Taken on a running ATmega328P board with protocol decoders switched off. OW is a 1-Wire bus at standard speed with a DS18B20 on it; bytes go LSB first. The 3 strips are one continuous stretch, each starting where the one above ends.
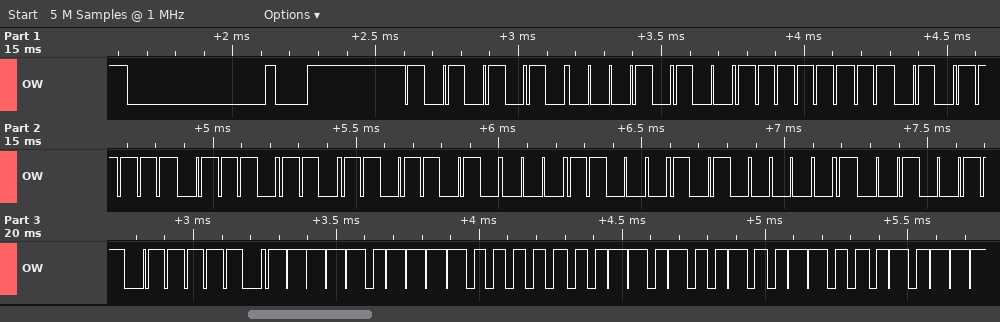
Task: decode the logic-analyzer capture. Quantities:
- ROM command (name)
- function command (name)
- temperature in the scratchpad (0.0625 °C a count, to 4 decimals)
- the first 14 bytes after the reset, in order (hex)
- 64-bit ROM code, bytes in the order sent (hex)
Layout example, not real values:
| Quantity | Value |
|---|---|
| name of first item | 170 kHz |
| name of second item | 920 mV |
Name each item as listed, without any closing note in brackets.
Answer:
| Quantity | Value |
|---|---|
| ROM command | Match ROM |
| function command | Read Scratchpad |
| temperature in the scratchpad | 30.9375 °C |
| the first 14 bytes after the reset, in order | 55 28 FF FA 6E 5B 18 05 C9 BE EF 01 4B 46 |
| 64-bit ROM code, bytes in the order sent | 28 FF FA 6E 5B 18 05 C9 |
